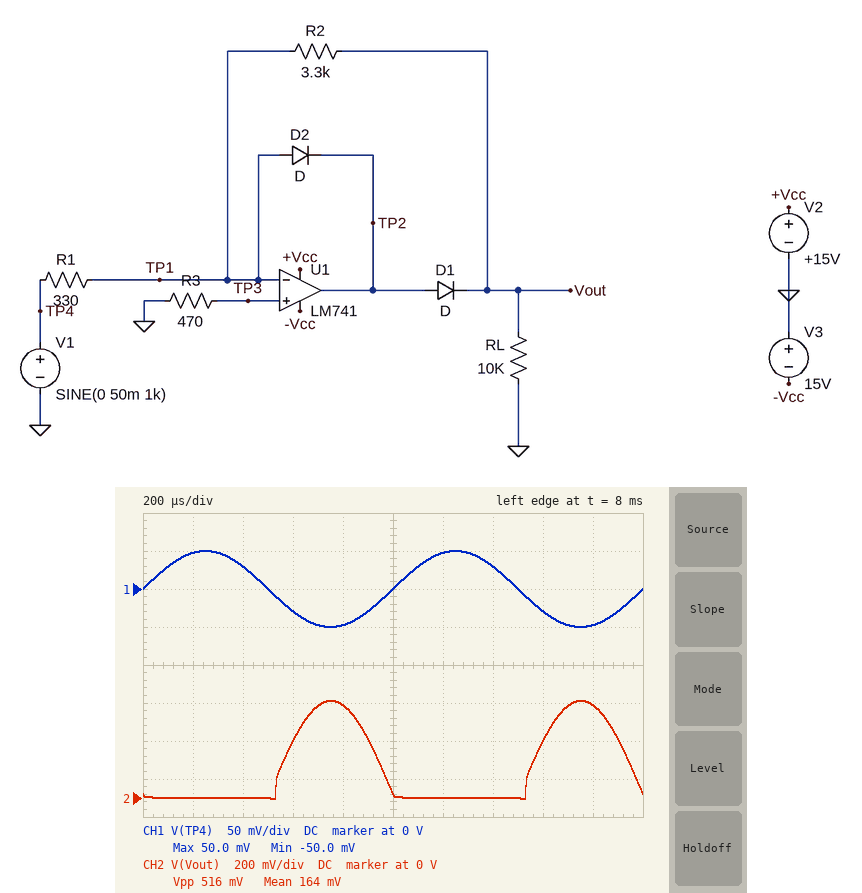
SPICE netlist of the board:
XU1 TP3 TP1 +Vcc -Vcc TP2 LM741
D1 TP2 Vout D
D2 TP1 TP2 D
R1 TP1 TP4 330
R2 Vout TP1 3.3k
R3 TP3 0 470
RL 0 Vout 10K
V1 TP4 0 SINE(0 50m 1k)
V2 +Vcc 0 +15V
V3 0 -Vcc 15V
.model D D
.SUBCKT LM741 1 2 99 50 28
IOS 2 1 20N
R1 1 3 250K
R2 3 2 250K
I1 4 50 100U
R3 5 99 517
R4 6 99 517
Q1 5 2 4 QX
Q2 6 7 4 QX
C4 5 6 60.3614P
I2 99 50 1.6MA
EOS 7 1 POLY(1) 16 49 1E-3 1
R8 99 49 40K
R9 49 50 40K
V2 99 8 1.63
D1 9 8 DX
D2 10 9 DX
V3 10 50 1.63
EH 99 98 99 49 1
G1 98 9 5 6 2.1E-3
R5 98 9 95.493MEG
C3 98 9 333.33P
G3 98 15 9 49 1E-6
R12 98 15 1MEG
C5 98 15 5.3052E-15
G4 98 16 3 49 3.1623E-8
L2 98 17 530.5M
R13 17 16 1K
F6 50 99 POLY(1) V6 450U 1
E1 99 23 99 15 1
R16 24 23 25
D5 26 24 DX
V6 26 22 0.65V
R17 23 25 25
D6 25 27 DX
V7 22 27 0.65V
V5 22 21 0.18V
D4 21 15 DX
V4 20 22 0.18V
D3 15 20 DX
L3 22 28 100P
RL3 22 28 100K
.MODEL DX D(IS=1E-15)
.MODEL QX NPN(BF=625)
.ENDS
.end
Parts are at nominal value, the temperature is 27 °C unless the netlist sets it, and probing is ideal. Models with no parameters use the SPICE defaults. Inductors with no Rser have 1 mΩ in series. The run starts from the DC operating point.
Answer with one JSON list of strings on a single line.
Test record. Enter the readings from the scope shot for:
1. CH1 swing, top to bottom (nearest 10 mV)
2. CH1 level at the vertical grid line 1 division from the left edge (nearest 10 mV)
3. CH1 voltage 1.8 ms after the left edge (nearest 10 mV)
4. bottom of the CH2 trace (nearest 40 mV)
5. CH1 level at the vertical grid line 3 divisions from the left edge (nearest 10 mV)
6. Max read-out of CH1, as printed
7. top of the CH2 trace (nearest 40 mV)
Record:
["100 mV", "50 mV", "-50 mV", "0 V", "-30 mV", "50.0 mV", "520 mV"]
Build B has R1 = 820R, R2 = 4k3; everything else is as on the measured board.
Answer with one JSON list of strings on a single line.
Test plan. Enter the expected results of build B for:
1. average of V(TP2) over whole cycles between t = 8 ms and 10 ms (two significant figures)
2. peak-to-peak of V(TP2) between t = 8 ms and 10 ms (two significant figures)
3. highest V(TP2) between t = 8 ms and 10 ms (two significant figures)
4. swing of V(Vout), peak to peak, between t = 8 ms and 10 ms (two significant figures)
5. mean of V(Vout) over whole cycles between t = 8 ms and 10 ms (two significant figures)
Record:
["100 mV", "1.4 V", "860 mV", "270 mV", "86 mV"]
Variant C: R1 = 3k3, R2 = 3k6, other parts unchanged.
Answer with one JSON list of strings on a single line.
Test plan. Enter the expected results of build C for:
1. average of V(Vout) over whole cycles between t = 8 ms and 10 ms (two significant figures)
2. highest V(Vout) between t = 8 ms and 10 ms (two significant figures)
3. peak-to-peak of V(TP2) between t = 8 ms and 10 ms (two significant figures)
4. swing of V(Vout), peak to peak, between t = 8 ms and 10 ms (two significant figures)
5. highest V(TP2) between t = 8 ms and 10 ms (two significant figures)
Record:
["19 mV", "57 mV", "1.2 V", "62 mV", "610 mV"]
